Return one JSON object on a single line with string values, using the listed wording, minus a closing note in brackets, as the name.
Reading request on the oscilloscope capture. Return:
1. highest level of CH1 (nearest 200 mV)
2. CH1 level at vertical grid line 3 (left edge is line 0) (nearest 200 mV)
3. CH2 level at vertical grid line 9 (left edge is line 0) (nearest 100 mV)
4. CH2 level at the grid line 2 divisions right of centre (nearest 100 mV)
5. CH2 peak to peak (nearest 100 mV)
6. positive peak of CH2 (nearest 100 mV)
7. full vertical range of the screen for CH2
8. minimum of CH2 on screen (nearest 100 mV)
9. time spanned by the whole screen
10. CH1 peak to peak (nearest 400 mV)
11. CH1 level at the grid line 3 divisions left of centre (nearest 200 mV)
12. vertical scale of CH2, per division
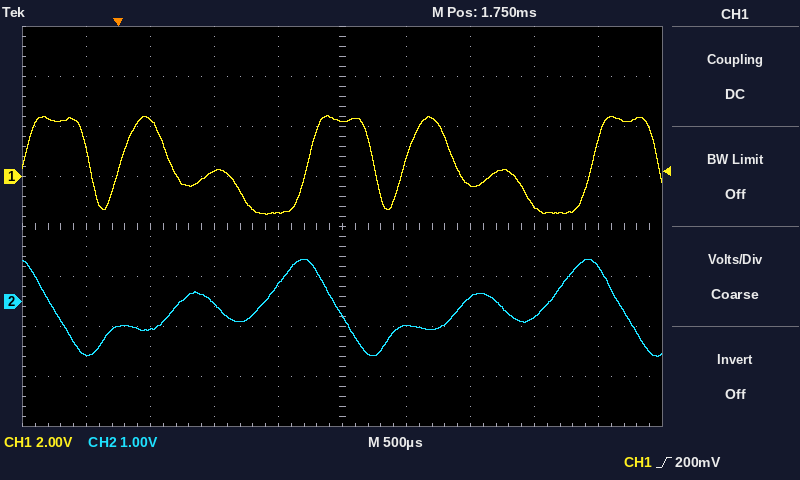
{"highest level of CH1": "2.4 V", "CH1 level at vertical grid line 3 (left edge is line 0)": "200 mV", "CH2 level at vertical grid line 9 (left edge is line 0)": "700 mV", "CH2 level at the grid line 2 divisions right of centre": "100 mV", "CH2 peak to peak": "1.9 V", "positive peak of CH2": "800 mV", "full vertical range of the screen for CH2": "8 V", "minimum of CH2 on screen": "-1.1 V", "time spanned by the whole screen": "5 ms", "CH1 peak to peak": "4.0 V", "CH1 level at the grid line 3 divisions left of centre": "2.2 V", "vertical scale of CH2, per division": "1 V"}
